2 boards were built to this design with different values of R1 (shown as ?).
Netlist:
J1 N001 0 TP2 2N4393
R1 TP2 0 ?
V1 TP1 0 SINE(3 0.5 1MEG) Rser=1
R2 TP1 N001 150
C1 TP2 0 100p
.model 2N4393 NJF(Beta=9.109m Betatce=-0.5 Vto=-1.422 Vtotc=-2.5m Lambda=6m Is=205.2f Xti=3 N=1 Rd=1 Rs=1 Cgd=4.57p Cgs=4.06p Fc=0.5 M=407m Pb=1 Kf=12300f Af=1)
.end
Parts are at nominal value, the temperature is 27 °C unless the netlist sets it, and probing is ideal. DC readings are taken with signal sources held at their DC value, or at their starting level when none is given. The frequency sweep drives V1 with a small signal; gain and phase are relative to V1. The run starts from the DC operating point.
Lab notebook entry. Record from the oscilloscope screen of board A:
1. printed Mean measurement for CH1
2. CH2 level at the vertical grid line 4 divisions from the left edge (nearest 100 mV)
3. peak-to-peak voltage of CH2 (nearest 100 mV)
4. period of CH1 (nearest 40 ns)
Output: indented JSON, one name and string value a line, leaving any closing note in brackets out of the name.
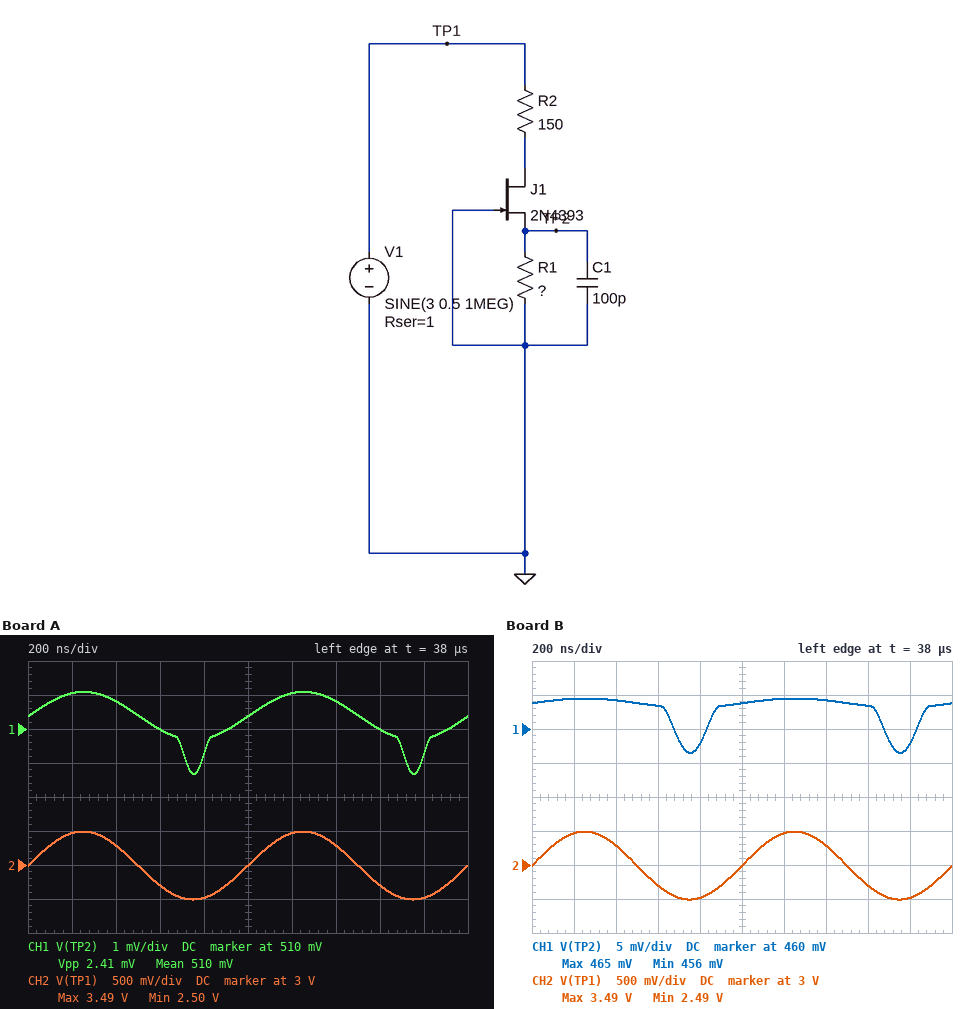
{
  "printed Mean measurement for CH1": "510 mV",
  "CH2 level at the vertical grid line 4 divisions from the left edge": "2.5 V",
  "peak-to-peak voltage of CH2": "1.0 V",
  "period of CH1": "1.00 µs"
}
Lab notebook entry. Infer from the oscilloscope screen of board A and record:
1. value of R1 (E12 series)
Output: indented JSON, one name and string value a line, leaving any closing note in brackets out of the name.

{
  "value of R1": "68 Ω"
}
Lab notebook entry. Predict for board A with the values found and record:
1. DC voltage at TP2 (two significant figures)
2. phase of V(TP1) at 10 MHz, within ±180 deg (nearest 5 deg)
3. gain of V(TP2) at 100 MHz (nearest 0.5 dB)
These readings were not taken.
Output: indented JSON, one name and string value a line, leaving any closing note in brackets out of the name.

{
  "DC voltage at TP2": "510 mV",
  "phase of V(TP1) at 10 MHz, within ±180 deg": "0 deg",
  "gain of V(TP2) at 100 MHz": "-64.5 dB"
}
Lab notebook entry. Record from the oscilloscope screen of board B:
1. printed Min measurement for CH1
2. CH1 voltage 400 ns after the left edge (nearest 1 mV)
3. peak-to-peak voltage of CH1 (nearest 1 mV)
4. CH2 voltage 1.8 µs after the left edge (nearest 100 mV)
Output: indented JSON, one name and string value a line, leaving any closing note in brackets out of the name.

{
  "printed Min measurement for CH1": "456 mV",
  "CH1 voltage 400 ns after the left edge": "464 mV",
  "peak-to-peak voltage of CH1": "8 mV",
  "CH2 voltage 1.8 µs after the left edge": "2.5 V"
}
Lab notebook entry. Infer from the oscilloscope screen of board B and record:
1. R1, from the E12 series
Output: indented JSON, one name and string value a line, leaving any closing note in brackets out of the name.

{
  "R1, from the E12 series": "56 Ω"
}
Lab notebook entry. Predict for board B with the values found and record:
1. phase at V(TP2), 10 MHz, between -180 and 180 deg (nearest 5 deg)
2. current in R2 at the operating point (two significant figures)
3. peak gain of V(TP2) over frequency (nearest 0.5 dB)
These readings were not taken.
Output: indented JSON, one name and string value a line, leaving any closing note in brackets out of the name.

{
  "phase at V(TP2), 10 MHz, between -180 and 180 deg": "-10 deg",
  "current in R2 at the operating point": "8.3 mA",
  "peak gain of V(TP2) over frequency": "-57.0 dB"
}
